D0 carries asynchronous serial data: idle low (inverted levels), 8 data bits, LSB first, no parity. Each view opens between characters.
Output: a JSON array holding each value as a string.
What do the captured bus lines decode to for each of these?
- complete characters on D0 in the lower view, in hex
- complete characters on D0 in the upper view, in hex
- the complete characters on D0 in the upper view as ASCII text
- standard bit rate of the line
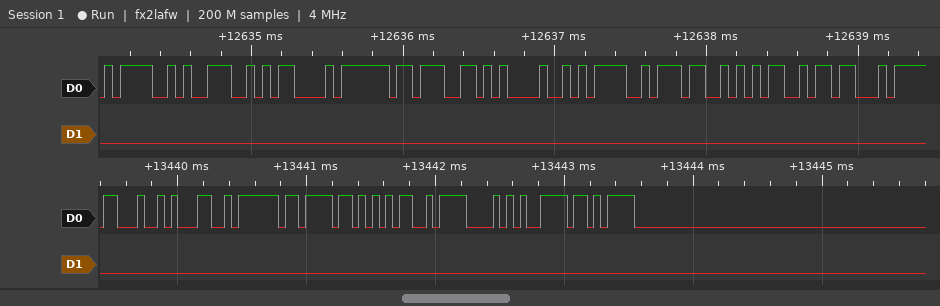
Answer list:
["6E, 67, 20, 48, 65, 78, 0D, 0A", "61, 63, 79, 20, 4C, 6F, 61, 64, 65, 72", "\"acy Loader\"", "19200 baud"]
